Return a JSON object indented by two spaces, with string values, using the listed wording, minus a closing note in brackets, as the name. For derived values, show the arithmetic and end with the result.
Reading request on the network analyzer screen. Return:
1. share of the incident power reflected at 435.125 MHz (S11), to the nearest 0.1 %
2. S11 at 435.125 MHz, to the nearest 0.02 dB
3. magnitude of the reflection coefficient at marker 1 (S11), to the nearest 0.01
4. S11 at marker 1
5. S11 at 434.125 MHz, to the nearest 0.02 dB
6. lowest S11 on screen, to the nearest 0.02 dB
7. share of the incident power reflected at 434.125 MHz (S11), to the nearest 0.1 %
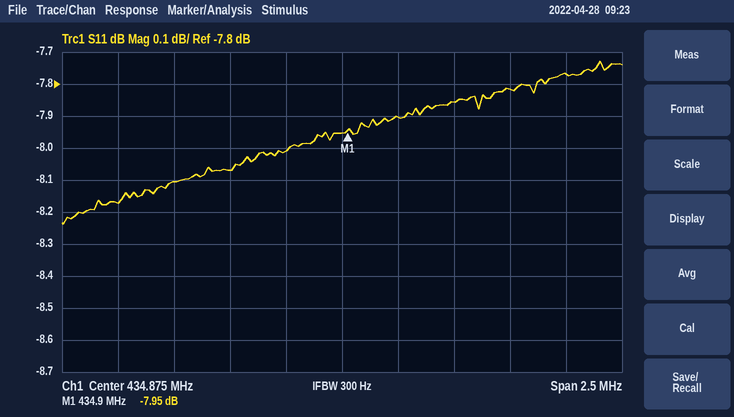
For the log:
{
  "share of the incident power reflected at 435.125 MHz (S11), to the nearest 0.1 %": "10^(-7.9/10) ≈ 16.2 %",
  "S11 at 435.125 MHz, to the nearest 0.02 dB": "-7.90 dB",
  "magnitude of the reflection coefficient at marker 1 (S11), to the nearest 0.01": "10^(-7.95/20) ≈ 0.40",
  "S11 at marker 1": "-7.95 dB",
  "S11 at 434.125 MHz, to the nearest 0.02 dB": "-8.10 dB",
  "lowest S11 on screen, to the nearest 0.02 dB": "-8.24 dB",
  "share of the incident power reflected at 434.125 MHz (S11), to the nearest 0.1 %": "10^(-8.1/10) ≈ 15.5 %"
}
